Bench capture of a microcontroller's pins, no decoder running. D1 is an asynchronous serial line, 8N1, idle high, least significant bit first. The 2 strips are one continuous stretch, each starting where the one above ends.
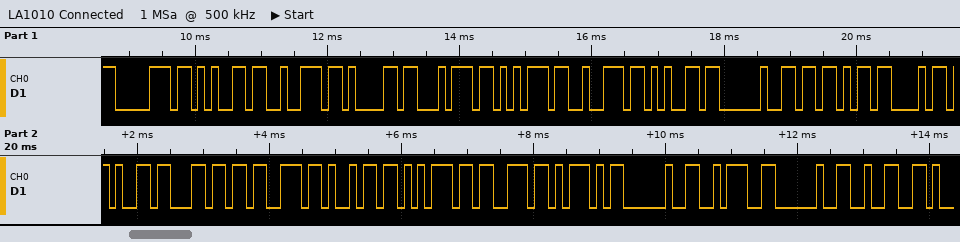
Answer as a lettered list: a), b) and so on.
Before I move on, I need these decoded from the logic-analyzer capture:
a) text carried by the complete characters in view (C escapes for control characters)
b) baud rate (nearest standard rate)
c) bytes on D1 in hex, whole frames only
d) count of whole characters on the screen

a) "perature [Celsius] : 2"
b) 9600 baud
c) 70 65 72 61 74 75 72 65 20 5B 43 65 6C 73 69 75 73 5D 20 3A 20 32
d) 22
